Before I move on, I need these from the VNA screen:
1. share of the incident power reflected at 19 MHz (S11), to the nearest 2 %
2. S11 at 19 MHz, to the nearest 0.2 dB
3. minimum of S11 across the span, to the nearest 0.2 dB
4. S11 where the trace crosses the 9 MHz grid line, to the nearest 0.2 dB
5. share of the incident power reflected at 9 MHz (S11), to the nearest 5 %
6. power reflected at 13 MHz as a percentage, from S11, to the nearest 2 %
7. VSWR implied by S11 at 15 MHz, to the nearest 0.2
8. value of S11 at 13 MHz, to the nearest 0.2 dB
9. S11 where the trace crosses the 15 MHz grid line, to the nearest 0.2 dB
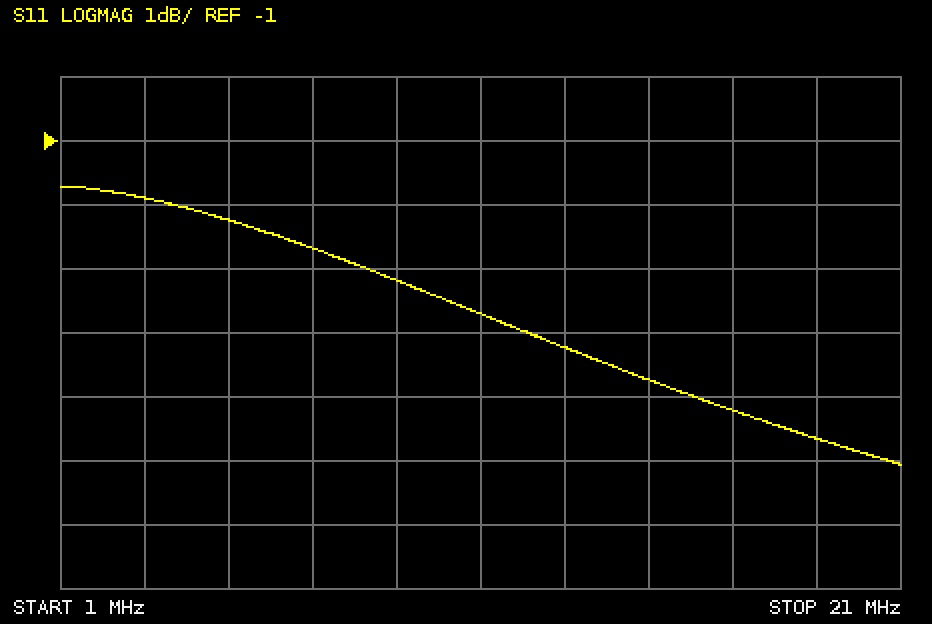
28 %
-5.6 dB
-6.0 dB
-3.2 dB
50 %
38 %
3.8
-4.2 dB
-4.8 dB
